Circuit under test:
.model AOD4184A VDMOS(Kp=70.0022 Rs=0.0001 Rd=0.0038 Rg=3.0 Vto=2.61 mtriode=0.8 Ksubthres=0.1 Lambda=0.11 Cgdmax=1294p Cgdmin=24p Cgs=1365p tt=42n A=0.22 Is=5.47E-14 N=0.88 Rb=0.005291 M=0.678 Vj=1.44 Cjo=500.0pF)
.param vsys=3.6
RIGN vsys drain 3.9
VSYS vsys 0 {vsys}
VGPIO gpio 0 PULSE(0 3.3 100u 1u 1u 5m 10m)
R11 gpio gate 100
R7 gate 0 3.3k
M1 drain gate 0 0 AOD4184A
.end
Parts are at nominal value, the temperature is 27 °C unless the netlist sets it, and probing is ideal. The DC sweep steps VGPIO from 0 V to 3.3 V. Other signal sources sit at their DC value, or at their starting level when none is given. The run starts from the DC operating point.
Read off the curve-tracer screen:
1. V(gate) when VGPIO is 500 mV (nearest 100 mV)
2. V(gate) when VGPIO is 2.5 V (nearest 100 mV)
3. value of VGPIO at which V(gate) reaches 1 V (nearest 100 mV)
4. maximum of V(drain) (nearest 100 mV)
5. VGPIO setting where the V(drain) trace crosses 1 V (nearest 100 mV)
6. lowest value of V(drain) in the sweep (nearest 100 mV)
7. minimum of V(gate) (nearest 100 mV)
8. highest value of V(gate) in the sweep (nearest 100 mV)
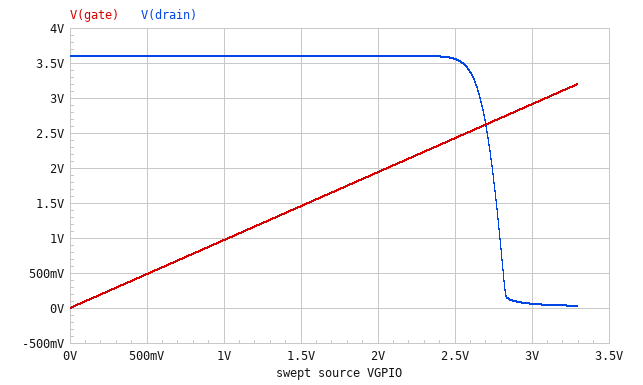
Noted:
500 mV
2.4 V
1.0 V
3.6 V
2.8 V
0 V
0 V
3.2 V
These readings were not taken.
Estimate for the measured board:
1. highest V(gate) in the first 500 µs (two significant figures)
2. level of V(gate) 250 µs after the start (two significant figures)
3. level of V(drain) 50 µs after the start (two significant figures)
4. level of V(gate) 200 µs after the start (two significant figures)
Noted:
3.2 V
3.2 V
3.6 V
3.2 V
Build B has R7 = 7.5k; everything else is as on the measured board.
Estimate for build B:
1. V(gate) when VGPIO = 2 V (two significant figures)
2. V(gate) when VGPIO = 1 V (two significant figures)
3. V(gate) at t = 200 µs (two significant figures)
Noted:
2.0 V
990 mV
3.3 V
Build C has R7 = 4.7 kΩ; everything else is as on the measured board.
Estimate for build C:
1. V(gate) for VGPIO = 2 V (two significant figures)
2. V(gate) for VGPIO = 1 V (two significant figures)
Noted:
2.0 V
980 mV
